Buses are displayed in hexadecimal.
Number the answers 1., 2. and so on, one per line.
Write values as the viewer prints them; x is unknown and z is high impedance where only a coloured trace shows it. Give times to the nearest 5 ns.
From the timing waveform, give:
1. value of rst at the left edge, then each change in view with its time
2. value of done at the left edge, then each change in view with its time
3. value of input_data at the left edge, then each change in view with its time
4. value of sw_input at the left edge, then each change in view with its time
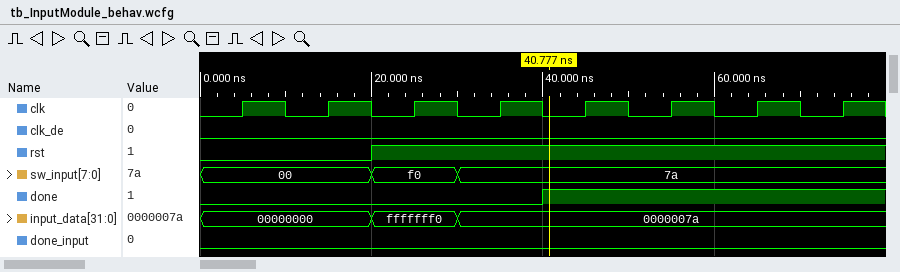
1. 0, 1 at 20 ns
2. 0, 1 at 40 ns
3. 00000000, fffffff0 at 20 ns, 0000007a at 30 ns
4. 00, f0 at 20 ns, 7a at 30 ns
